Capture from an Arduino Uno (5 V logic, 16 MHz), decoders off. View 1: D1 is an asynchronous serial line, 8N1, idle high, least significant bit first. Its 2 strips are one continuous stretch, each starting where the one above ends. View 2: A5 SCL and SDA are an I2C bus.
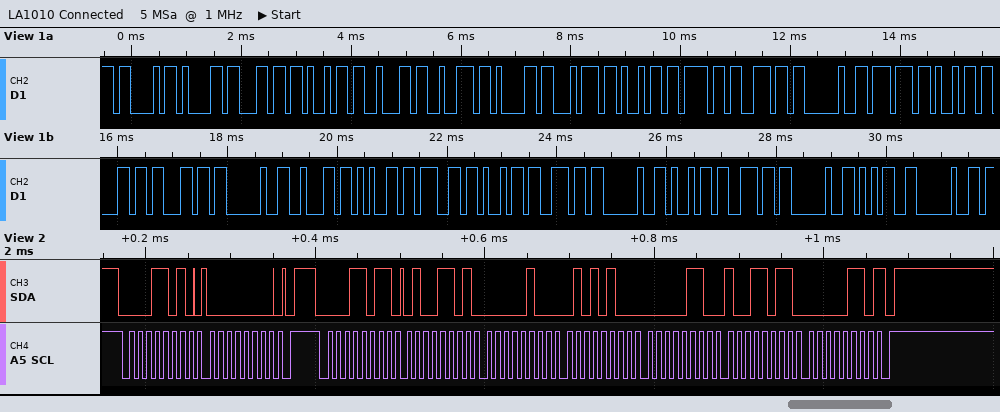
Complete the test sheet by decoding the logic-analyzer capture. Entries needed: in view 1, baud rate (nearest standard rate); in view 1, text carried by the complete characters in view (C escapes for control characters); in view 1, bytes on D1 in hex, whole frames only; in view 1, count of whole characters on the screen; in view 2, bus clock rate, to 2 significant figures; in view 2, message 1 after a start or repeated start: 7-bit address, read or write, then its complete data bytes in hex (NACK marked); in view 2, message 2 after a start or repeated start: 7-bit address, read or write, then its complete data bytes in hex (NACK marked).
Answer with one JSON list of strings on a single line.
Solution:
["9600 baud", "\"Calibration will begin in 5 \"", "43 61 6C 69 62 72 61 74 69 6F 6E 20 77 69 6C 6C 20 62 65 67 69 6E 20 69 6E 20 35 20", "28", "100 kHz", "0x0D write: 00", "0x0D read: 4D 04 54 06 9B 06 NACK"]
